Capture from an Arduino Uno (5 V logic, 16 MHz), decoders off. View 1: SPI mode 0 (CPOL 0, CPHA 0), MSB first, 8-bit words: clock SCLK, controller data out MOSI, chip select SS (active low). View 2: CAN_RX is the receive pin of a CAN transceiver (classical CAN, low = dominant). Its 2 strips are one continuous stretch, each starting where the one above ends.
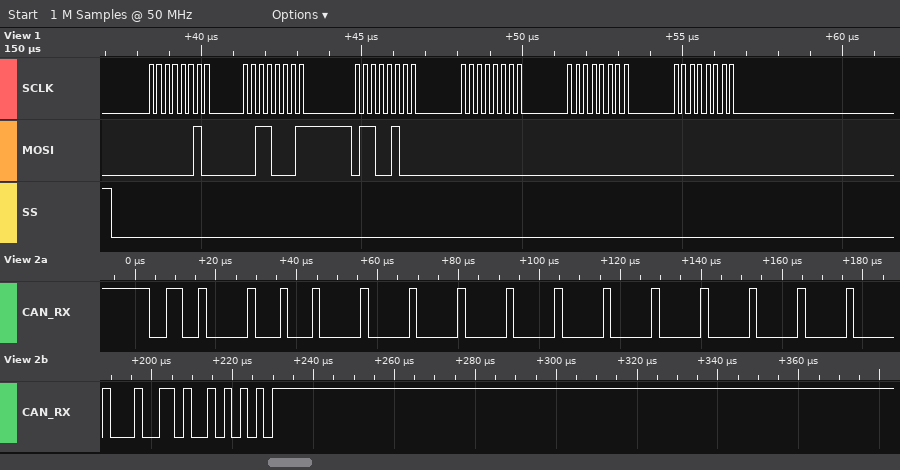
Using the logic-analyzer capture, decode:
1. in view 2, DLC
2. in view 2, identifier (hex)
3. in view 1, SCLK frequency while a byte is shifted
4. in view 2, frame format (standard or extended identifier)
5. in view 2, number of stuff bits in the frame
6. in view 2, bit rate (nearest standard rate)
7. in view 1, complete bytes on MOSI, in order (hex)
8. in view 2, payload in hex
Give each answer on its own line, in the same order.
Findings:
8
0x320
4 MHz
standard
13
500 kbit/s
02 31 64 00 00 00
80 00 00 00 00 00 00 00
